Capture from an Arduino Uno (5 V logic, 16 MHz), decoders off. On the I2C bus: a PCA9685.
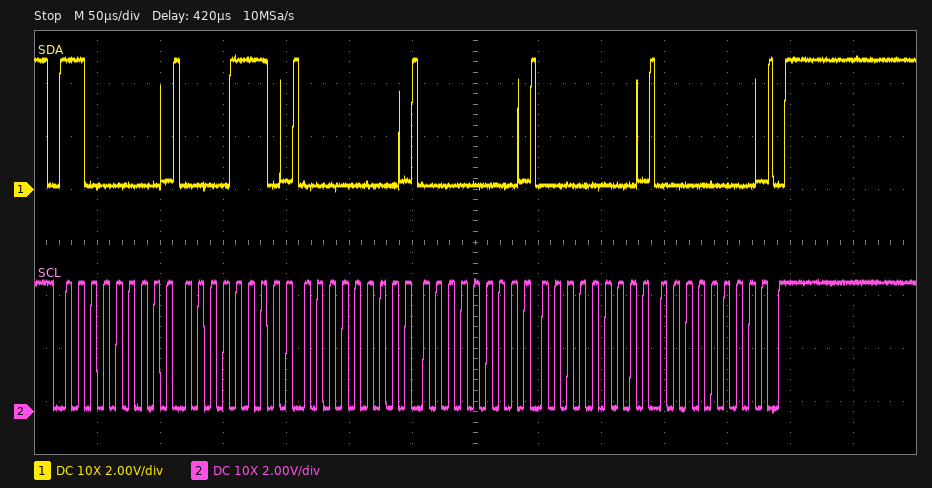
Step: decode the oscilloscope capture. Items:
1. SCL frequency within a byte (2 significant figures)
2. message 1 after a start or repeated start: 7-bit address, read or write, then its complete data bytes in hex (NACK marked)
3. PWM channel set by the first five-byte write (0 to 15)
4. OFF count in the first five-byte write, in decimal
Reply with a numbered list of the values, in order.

1. 100 kHz
2. 0x60 write: 0E 00 00 00 00
3. 2
4. 0
